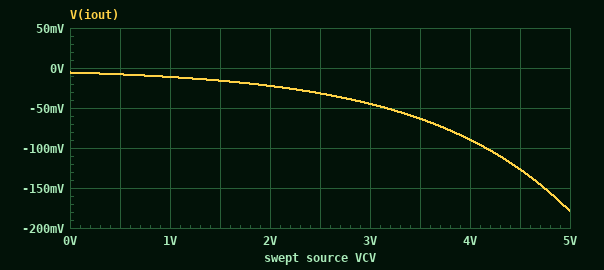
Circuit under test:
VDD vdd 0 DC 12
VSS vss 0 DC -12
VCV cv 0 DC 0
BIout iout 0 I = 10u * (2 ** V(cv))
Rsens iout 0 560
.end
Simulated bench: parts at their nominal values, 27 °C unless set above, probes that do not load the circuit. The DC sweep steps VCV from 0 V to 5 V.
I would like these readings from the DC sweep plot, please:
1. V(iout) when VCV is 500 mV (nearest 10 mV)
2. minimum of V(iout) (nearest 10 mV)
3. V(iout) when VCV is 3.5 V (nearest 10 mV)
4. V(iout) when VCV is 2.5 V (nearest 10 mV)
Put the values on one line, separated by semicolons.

-10 mV; -180 mV; -60 mV; -30 mV
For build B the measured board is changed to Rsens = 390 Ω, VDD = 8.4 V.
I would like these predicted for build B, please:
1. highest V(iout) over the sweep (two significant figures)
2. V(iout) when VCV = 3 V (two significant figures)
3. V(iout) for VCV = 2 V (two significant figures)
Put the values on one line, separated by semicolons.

-3.9 mV; -31 mV; -16 mV
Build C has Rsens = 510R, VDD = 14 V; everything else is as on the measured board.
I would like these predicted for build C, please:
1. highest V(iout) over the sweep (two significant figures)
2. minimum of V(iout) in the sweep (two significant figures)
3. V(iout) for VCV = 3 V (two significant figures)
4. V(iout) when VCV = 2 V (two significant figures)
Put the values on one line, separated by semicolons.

-5.1 mV; -160 mV; -41 mV; -20 mV
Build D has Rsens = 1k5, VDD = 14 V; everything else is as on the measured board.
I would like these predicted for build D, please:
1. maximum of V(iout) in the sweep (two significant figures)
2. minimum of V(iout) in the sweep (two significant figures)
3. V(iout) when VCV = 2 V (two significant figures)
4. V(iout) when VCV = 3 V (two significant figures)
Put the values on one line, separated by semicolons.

-15 mV; -480 mV; -60 mV; -120 mV
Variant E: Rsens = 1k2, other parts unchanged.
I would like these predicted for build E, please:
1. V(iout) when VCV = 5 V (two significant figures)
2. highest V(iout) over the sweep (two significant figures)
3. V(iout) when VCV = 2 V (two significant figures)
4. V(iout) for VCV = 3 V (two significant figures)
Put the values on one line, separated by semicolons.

-380 mV; -12 mV; -48 mV; -96 mV
